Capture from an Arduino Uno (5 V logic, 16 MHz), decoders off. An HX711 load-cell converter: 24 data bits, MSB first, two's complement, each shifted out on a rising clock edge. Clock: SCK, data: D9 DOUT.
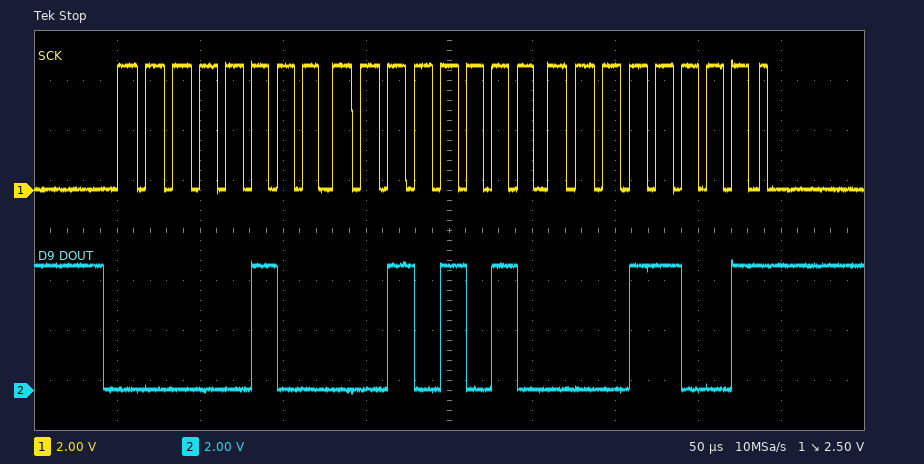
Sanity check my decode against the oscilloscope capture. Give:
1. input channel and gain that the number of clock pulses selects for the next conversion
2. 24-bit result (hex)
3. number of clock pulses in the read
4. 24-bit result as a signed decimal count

channel A, gain 128
0x042A19
25
272921
